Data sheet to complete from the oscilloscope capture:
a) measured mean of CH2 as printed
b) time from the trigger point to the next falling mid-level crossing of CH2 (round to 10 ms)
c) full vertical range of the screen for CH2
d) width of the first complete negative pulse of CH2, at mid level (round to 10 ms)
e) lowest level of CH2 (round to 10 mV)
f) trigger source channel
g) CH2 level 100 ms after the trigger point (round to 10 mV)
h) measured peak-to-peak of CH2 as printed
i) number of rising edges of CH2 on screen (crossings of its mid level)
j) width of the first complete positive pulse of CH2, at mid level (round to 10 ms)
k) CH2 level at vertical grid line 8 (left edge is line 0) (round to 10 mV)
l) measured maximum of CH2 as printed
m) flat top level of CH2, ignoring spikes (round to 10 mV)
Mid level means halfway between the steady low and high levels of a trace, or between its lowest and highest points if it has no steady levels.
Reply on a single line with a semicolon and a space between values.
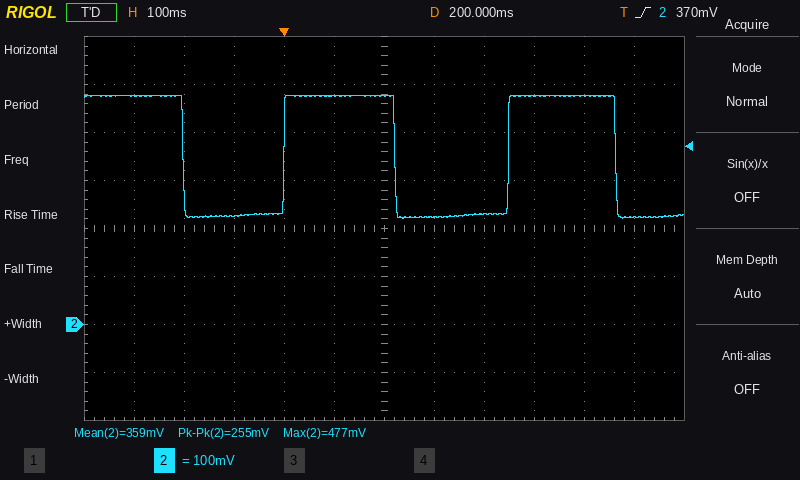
359 mV; 220 ms; 800 mV; 200 ms; 220 mV; CH2; 480 mV; 255 mV; 2; 220 ms; 230 mV; 477 mV; 480 mV
